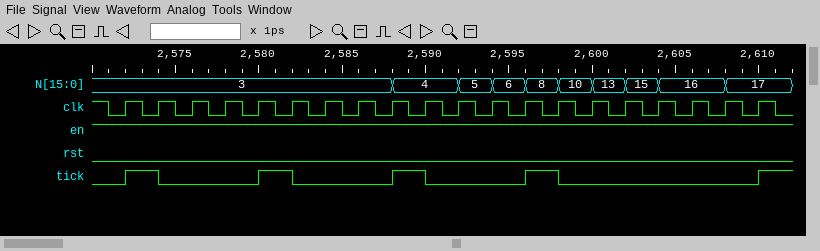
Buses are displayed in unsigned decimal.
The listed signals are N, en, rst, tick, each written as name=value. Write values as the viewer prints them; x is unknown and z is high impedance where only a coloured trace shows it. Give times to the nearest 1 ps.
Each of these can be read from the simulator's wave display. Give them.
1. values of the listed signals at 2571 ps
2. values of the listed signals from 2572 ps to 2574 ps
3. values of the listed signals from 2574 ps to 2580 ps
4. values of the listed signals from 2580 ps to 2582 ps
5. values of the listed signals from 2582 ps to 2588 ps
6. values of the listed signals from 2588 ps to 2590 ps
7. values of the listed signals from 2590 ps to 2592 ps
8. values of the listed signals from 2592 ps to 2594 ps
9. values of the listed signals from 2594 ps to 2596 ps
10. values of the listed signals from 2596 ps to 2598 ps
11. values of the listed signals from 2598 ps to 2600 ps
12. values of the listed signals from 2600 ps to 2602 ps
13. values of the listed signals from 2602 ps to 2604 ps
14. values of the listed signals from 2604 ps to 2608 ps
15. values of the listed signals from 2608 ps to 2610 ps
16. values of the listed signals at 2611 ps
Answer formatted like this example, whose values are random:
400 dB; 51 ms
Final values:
N=3, en=1, rst=0, tick=0; N=3, en=1, rst=0, tick=1; N=3, en=1, rst=0, tick=0; N=3, en=1, rst=0, tick=1; N=3, en=1, rst=0, tick=0; N=4, en=1, rst=0, tick=1; N=4, en=1, rst=0, tick=0; N=5, en=1, rst=0, tick=0; N=6, en=1, rst=0, tick=0; N=8, en=1, rst=0, tick=1; N=10, en=1, rst=0, tick=0; N=13, en=1, rst=0, tick=0; N=15, en=1, rst=0, tick=0; N=16, en=1, rst=0, tick=0; N=17, en=1, rst=0, tick=0; N=17, en=1, rst=0, tick=1
